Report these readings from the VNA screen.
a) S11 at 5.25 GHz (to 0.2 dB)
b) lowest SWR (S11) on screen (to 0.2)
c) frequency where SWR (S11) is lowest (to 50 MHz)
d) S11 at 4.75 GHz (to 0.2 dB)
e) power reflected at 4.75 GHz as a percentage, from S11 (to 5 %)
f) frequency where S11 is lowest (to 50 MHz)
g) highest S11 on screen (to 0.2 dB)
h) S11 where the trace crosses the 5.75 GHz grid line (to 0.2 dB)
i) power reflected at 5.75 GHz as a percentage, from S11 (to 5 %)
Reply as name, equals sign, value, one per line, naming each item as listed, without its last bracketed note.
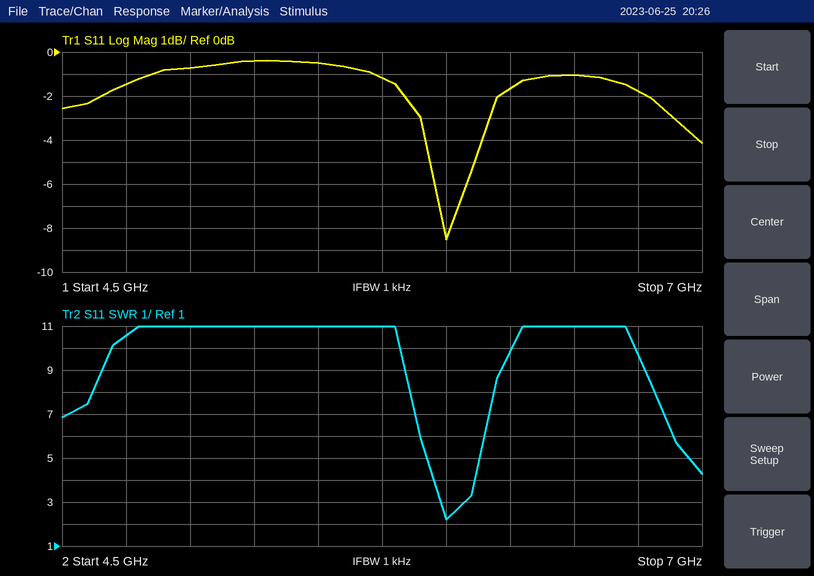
S11 at 5.25 GHz = -0.4 dB
lowest SWR (S11) on screen = 2.2
frequency where SWR (S11) is lowest = 6.00 GHz
S11 at 4.75 GHz = -1.4 dB
power reflected at 4.75 GHz as a percentage, from S11 = 70 %
frequency where S11 is lowest = 6.00 GHz
highest S11 on screen = -0.4 dB
S11 where the trace crosses the 5.75 GHz grid line = -1.2 dB
power reflected at 5.75 GHz as a percentage, from S11 = 75 %
